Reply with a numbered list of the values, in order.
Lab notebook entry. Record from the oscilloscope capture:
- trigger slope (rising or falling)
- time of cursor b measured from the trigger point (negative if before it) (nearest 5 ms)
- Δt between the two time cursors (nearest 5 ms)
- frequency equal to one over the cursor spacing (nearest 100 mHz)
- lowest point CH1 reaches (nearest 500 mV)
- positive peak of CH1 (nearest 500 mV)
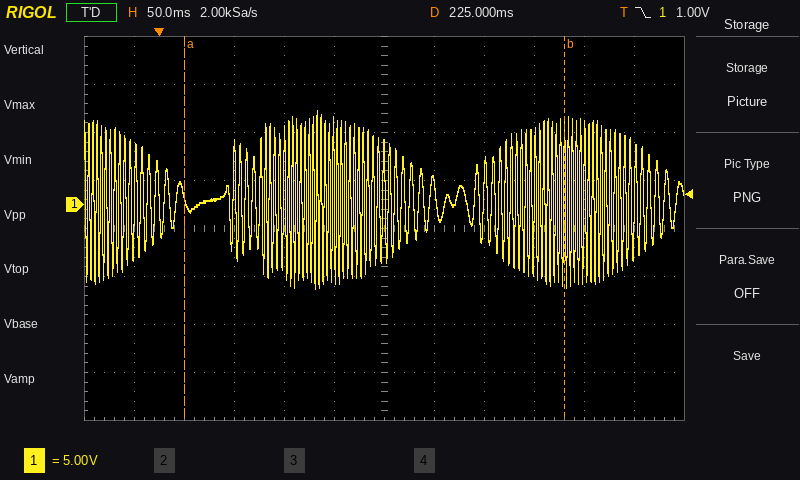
1. falling
2. +405 ms
3. 380 ms
4. 2.6 Hz
5. -9.0 V
6. 10.0 V
